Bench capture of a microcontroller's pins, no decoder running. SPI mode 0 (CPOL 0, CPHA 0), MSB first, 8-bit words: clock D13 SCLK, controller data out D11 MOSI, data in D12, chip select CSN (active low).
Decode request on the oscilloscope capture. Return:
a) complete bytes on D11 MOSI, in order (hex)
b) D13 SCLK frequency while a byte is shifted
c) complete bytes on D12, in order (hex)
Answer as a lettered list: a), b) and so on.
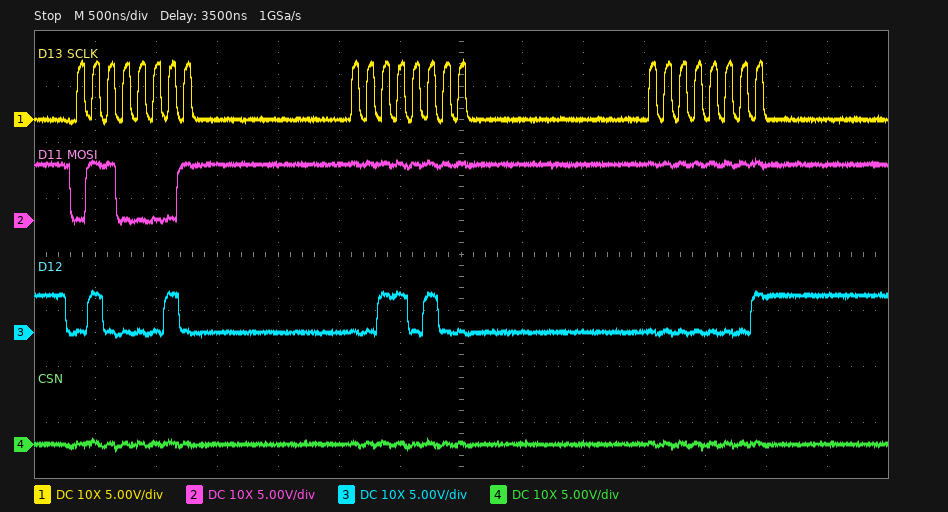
a) 61 FF FF
b) 8 MHz
c) 42 34 01
